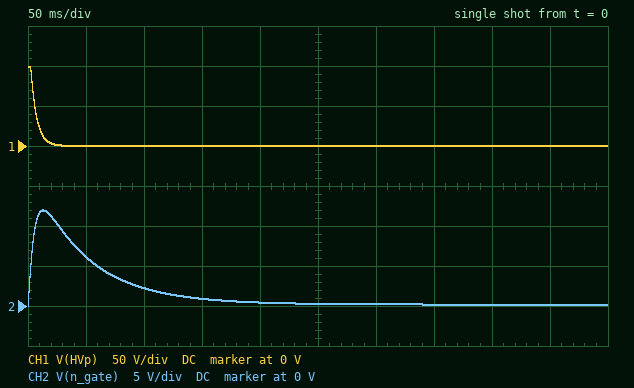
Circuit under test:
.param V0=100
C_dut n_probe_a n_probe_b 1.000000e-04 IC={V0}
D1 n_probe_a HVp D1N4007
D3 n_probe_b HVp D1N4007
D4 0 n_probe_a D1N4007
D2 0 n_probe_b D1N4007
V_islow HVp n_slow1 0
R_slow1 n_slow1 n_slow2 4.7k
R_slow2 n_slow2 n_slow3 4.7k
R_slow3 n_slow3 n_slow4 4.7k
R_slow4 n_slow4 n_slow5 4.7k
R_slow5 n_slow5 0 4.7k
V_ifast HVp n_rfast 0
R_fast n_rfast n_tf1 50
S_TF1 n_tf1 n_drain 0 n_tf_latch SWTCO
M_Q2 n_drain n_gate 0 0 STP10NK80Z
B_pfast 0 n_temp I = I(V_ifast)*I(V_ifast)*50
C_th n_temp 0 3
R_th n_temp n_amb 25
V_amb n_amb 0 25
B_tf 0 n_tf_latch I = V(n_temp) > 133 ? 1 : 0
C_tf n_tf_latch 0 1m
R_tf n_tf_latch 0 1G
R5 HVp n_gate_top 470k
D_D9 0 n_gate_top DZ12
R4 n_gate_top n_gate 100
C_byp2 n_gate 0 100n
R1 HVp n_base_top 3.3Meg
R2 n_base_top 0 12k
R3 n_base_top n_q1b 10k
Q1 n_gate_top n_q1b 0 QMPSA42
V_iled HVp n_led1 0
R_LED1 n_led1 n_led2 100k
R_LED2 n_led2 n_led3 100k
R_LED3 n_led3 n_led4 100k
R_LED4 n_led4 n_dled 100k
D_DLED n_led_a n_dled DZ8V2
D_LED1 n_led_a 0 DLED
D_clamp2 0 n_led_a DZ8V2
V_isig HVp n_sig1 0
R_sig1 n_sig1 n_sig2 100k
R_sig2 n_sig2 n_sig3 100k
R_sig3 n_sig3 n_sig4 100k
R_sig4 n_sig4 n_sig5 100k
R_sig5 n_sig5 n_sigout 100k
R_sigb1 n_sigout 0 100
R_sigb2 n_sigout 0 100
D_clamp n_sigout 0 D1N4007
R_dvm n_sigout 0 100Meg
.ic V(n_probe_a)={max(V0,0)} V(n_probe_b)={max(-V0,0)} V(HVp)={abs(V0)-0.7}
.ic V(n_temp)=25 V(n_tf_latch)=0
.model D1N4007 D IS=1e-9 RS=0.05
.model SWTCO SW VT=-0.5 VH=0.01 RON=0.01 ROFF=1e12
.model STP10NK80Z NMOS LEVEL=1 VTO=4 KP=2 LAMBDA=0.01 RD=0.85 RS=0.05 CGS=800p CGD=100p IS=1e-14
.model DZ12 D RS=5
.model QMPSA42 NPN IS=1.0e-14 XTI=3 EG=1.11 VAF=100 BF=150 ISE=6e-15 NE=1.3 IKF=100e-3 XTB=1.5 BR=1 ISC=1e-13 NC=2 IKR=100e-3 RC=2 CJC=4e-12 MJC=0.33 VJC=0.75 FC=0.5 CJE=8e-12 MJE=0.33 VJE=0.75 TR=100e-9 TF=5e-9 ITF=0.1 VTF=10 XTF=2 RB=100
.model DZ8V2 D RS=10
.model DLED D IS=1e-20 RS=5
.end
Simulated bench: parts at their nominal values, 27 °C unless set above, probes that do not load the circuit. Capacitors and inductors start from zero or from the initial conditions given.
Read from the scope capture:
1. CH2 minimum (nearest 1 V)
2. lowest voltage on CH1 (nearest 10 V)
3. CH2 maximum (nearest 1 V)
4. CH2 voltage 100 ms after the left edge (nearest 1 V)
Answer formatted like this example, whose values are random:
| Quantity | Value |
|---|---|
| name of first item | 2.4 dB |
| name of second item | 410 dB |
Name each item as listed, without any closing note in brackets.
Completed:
| Quantity | Value |
|---|---|
| CH2 minimum | 0 V |
| lowest voltage on CH1 | 0 V |
| CH2 maximum | 12 V |
| CH2 voltage 100 ms after the left edge | 2 V |
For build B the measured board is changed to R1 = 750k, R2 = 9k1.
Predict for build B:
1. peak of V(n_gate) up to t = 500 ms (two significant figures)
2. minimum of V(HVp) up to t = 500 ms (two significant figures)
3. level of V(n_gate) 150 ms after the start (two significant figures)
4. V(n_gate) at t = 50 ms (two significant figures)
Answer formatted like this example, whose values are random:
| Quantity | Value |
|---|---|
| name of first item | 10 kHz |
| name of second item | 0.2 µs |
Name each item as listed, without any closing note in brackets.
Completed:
| Quantity | Value |
|---|---|
| peak of V(n_gate) up to t = 500 ms | 67 mV |
| minimum of V(HVp) up to t = 500 ms | 78 V |
| level of V(n_gate) 150 ms after the start | 61 mV |
| V(n_gate) at t = 50 ms | 60 mV |
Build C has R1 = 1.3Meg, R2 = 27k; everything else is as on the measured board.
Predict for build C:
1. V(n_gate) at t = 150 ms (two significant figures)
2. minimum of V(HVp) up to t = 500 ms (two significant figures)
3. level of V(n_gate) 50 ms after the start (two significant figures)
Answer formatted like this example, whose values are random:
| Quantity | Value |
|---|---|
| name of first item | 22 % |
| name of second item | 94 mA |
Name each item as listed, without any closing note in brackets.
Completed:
| Quantity | Value |
|---|---|
| V(n_gate) at t = 150 ms | 55 mV |
| minimum of V(HVp) up to t = 500 ms | 78 V |
| level of V(n_gate) 50 ms after the start | 54 mV |
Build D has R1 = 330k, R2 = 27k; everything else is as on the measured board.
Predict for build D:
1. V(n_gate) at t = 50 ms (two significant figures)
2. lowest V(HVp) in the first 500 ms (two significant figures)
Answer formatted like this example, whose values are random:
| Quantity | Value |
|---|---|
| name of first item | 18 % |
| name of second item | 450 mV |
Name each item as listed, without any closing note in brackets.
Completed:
| Quantity | Value |
|---|---|
| V(n_gate) at t = 50 ms | 30 mV |
| lowest V(HVp) in the first 500 ms | 77 V |
